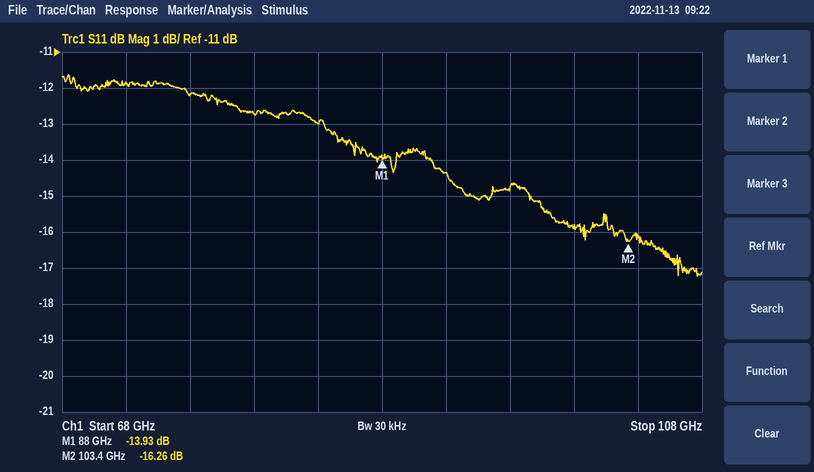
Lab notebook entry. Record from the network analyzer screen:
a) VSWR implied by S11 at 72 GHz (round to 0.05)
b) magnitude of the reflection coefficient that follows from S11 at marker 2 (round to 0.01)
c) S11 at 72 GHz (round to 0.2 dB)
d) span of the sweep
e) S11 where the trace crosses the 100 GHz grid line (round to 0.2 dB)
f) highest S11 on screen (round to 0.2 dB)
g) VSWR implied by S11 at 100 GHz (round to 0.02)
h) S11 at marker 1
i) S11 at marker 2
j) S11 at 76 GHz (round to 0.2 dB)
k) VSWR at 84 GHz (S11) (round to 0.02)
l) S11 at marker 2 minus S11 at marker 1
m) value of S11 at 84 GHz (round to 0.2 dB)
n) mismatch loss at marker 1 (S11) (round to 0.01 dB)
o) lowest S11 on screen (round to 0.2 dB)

1.70
0.15
-11.8 dB
40 GHz
-15.8 dB
-11.6 dB
1.38
-13.93 dB
-16.26 dB
-12.2 dB
1.58
-2.33 dB
-13.0 dB
0.18 dB
-17.2 dB
